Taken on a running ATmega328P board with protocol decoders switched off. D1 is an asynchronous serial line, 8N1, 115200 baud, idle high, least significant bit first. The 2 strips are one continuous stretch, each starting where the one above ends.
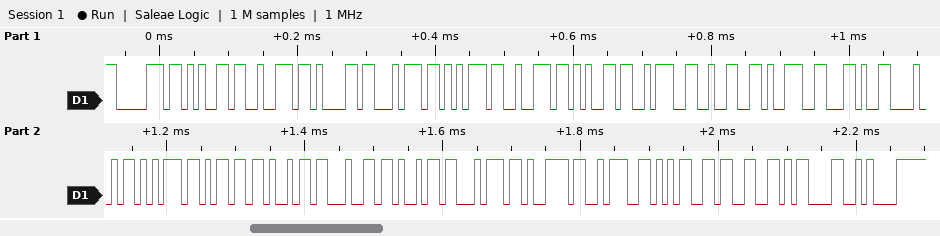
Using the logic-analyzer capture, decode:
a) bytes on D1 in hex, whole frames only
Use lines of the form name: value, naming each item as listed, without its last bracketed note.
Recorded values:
bytes on D1 in hex, whole frames only: 70 65 72 61 74 75 72 65 3A 32 39 2C 48 75 6D 69 64 69 74 79 3A 35 33 0D 0A
